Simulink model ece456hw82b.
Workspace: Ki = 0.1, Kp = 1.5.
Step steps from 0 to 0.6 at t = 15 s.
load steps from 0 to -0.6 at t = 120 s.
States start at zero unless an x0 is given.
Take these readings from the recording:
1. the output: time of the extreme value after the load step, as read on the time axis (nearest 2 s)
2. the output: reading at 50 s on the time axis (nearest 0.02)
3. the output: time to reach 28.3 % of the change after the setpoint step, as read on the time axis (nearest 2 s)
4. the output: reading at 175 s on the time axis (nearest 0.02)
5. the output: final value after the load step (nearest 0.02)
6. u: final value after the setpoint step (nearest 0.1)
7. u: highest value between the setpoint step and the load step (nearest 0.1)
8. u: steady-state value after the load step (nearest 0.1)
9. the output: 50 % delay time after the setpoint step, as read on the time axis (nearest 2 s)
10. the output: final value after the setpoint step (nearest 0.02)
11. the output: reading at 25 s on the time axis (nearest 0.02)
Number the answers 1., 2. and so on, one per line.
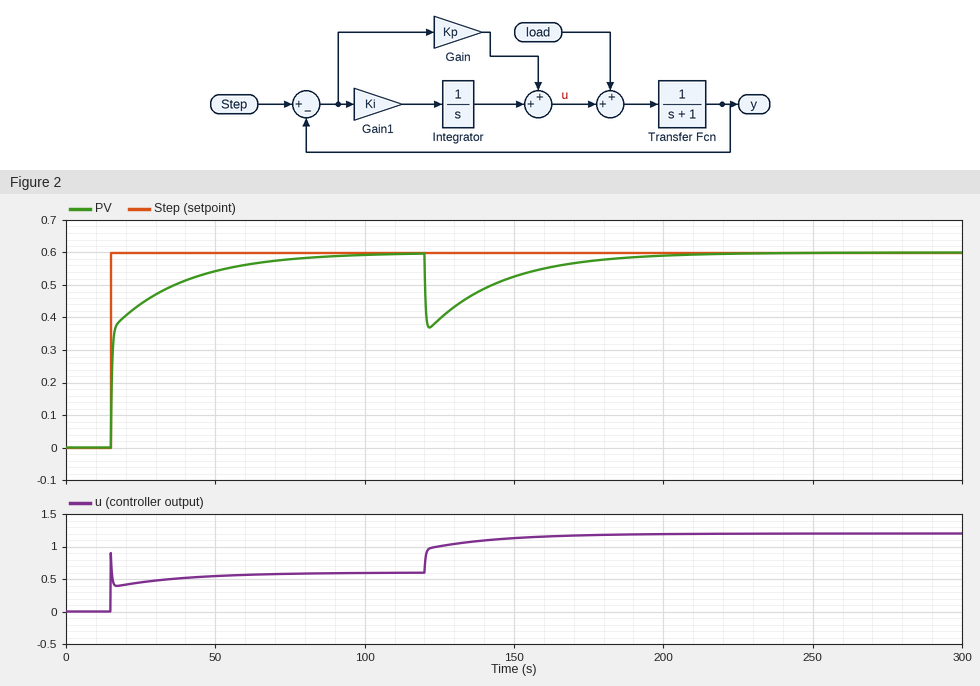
1. 122 s
2. 0.54
3. 16 s
4. 0.58
5. 0.60
6. 0.6
7. 0.9
8. 1.2
9. 16 s
10. 0.60
11. 0.44
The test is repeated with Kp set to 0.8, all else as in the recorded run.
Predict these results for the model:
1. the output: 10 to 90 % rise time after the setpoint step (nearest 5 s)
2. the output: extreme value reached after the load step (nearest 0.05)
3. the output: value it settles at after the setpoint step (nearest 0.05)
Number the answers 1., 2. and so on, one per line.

1. 30 s
2. 0.30
3. 0.60
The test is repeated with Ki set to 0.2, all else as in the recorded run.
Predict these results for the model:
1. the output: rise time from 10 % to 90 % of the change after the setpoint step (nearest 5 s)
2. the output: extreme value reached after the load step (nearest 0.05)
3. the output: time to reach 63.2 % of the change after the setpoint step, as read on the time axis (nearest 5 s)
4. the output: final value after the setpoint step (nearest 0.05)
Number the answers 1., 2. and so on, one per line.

1. 15 s
2. 0.40
3. 15 s
4. 0.60
